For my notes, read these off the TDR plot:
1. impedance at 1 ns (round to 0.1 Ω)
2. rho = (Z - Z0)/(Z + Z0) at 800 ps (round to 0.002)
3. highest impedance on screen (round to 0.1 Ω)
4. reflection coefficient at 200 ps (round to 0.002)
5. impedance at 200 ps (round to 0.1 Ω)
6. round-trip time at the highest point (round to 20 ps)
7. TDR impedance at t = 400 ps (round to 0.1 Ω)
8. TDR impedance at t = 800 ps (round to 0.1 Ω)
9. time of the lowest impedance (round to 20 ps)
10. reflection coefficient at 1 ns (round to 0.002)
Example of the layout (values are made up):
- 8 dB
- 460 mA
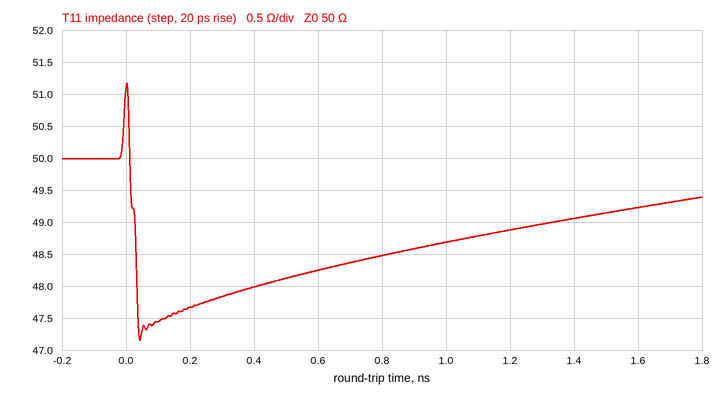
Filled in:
- 48.7 Ω
- -0.016
- 51.2 Ω
- -0.024
- 47.7 Ω
- 0 ps
- 48.0 Ω
- 48.5 Ω
- 40 ps
- -0.014
